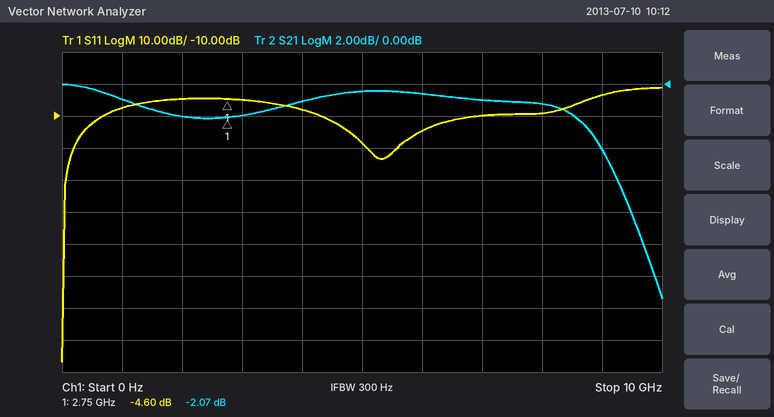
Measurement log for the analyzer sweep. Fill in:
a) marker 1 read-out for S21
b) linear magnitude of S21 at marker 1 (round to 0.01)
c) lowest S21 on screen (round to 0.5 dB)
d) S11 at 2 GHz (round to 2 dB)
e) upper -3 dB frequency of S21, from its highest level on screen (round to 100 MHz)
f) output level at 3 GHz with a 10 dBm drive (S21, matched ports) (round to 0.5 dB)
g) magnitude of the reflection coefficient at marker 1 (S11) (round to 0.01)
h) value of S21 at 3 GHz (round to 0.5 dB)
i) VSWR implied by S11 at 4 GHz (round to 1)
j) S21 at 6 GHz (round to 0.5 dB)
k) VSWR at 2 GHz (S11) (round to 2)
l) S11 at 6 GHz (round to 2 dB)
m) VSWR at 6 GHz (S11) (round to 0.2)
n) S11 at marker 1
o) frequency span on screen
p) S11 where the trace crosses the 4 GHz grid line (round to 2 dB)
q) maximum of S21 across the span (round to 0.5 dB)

-2.07 dB
0.79
-13.5 dB
-4 dB
8.8 GHz
8.0 dBm
0.59
-2.0 dB
2
-0.5 dB
4
-14 dB
1.4
-4.60 dB
10 GHz
-8 dB
0.0 dB
